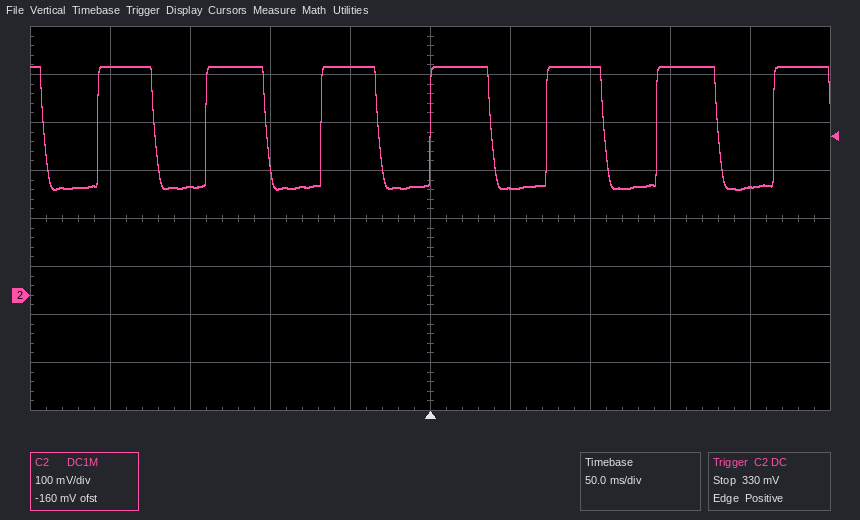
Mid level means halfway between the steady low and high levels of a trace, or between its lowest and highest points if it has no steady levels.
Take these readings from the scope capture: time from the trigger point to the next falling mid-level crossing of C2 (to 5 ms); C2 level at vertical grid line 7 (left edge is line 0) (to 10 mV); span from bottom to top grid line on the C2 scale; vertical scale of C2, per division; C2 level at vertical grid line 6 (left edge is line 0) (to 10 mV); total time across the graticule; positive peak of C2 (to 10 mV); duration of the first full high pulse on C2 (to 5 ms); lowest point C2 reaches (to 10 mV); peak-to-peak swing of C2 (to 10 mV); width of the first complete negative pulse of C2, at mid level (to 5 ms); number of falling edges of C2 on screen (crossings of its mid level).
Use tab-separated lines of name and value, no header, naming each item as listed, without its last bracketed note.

time from the trigger point to the next falling mid-level crossing of C2	40 ms
C2 level at vertical grid line 7 (left edge is line 0)	480 mV
span from bottom to top grid line on the C2 scale	800 mV
vertical scale of C2, per division	100 mV
C2 level at vertical grid line 6 (left edge is line 0)	220 mV
total time across the graticule	500 ms
positive peak of C2	480 mV
duration of the first full high pulse on C2	35 ms
lowest point C2 reaches	220 mV
peak-to-peak swing of C2	260 mV
width of the first complete negative pulse of C2, at mid level	35 ms
number of falling edges of C2 on screen	7
